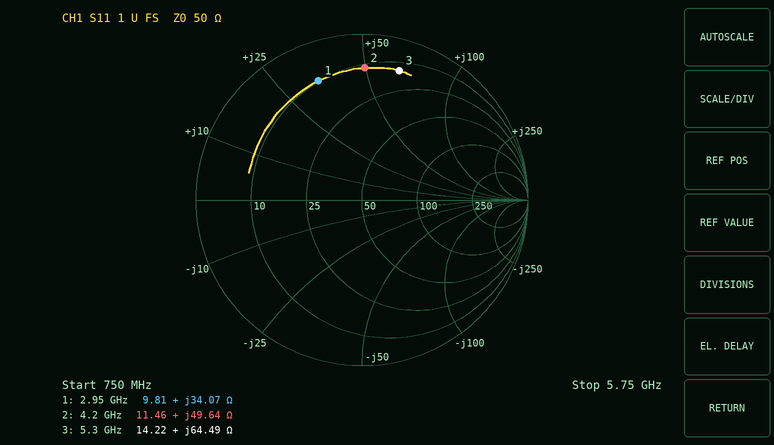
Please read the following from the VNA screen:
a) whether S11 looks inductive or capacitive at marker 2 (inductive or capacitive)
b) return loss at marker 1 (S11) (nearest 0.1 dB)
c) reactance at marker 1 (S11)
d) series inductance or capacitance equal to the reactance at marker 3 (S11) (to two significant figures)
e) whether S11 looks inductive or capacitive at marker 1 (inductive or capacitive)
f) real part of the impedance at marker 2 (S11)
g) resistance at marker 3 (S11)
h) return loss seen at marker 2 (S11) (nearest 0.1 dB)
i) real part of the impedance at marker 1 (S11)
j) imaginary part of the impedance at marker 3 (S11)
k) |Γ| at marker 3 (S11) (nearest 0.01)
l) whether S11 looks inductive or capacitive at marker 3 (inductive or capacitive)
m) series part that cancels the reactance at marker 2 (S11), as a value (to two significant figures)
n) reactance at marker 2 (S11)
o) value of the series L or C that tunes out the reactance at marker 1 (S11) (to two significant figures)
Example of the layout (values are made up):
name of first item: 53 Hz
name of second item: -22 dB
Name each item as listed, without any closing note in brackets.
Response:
whether S11 looks inductive or capacitive at marker 2: inductive
return loss at marker 1 (S11): 2.3 dB
reactance at marker 1: +34.07 Ω
series inductance or capacitance equal to the reactance at marker 3 (S11): 1.9 nH
whether S11 looks inductive or capacitive at marker 1: inductive
real part of the impedance at marker 2: 11.46 Ω
resistance at marker 3: 14.22 Ω
return loss seen at marker 2 (S11): 2.0 dB
real part of the impedance at marker 1: 9.81 Ω
imaginary part of the impedance at marker 3: +64.49 Ω
|Γ| at marker 3 (S11): 0.81
whether S11 looks inductive or capacitive at marker 3: inductive
series part that cancels the reactance at marker 2 (S11), as a value: 760 fF
reactance at marker 2: +49.64 Ω
value of the series L or C that tunes out the reactance at marker 1 (S11): 1.6 pF
